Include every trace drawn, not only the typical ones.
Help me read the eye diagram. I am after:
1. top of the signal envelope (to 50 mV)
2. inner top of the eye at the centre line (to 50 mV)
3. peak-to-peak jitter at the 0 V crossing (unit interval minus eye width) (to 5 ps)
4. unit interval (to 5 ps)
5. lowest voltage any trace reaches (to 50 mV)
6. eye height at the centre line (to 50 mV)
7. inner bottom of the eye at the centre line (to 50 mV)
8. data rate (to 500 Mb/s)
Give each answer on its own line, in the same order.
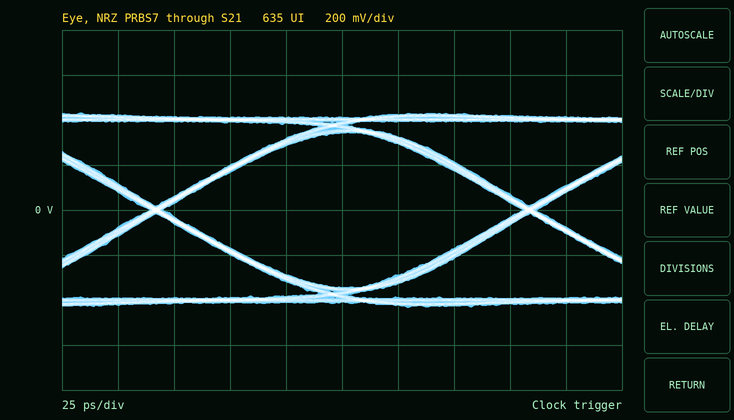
450 mV
350 mV
5 ps
165 ps
-450 mV
700 mV
-350 mV
6.0 Gb/s
